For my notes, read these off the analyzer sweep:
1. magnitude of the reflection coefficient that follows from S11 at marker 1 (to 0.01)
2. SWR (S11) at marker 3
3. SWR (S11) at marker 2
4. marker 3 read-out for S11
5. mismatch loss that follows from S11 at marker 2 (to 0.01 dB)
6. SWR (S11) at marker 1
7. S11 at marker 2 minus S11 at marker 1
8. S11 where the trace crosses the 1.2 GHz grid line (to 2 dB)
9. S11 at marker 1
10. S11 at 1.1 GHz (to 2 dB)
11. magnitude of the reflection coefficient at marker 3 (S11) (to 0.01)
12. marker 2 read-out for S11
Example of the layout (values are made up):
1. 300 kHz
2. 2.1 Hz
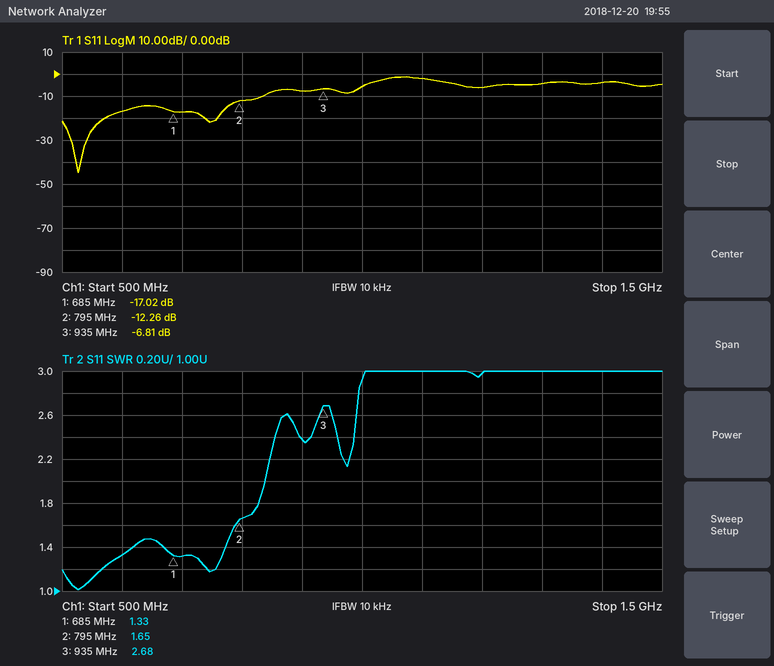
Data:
1. 0.14
2. 2.68
3. 1.65
4. -6.81 dB
5. 0.27 dB
6. 1.33
7. 4.76 dB
8. -6 dB
9. -17.02 dB
10. -2 dB
11. 0.46
12. -12.26 dB
